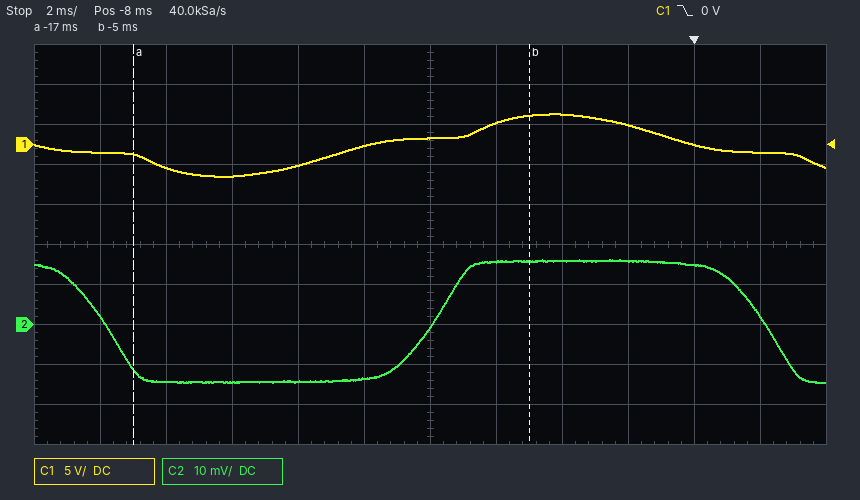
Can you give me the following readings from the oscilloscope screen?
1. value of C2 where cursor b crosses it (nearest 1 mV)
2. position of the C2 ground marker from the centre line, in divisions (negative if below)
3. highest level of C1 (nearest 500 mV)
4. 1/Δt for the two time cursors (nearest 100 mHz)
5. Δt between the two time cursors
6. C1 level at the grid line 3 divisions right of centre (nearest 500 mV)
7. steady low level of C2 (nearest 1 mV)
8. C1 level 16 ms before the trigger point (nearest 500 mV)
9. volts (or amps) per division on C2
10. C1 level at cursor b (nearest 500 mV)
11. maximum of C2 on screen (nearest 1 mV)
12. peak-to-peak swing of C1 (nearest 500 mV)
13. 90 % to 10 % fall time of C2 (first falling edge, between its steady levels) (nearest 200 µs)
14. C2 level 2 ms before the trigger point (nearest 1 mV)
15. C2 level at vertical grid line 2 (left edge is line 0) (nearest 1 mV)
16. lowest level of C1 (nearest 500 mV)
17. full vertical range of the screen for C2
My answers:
16 mV
-2.0 div
4.0 V
83.3 Hz
12.0 ms
2.5 V
-14 mV
-3.0 V
10 mV
3.5 V
16 mV
8.0 V
2.2 ms
16 mV
-14 mV
-4.0 V
100 mV
